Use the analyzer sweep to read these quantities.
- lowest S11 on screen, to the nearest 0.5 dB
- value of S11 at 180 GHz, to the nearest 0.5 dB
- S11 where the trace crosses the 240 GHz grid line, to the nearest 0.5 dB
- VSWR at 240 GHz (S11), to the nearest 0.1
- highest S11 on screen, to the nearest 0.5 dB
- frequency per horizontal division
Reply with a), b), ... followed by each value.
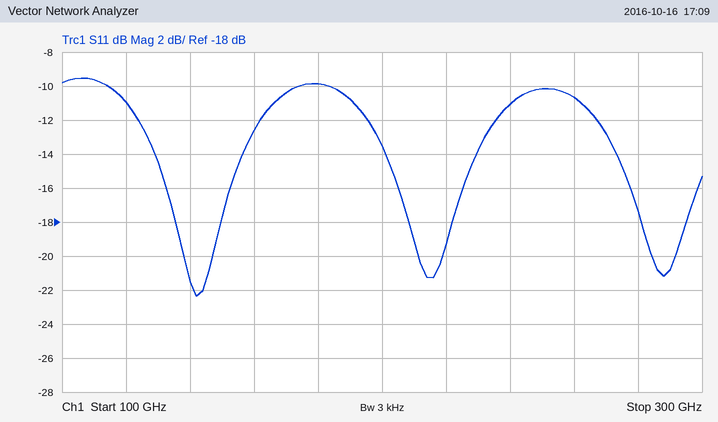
a) -22.5 dB
b) -10.0 dB
c) -11.0 dB
d) 1.8
e) -9.5 dB
f) 20 GHz
